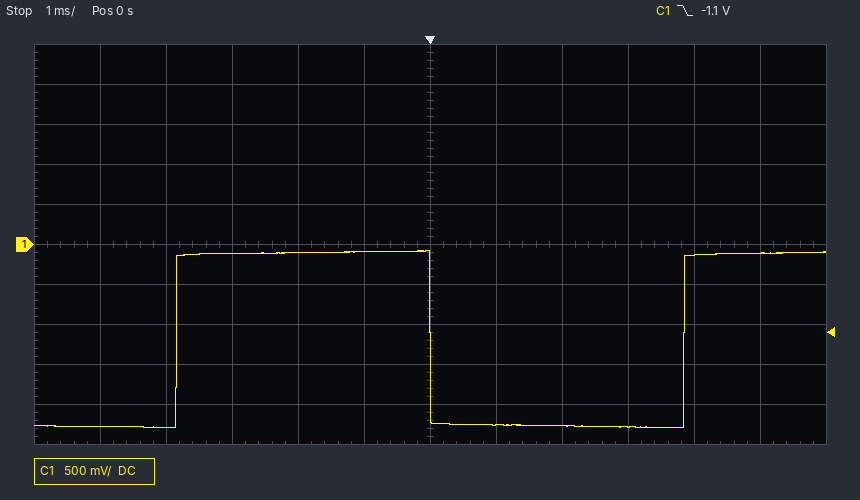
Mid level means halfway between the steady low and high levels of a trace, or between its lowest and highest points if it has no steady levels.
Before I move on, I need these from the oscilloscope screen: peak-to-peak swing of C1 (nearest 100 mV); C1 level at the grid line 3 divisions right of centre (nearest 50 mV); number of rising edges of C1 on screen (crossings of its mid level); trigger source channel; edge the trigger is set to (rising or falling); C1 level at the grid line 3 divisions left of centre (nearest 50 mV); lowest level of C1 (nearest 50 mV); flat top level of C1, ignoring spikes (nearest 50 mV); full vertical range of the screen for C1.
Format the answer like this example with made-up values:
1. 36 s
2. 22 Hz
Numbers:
1. 2.20 V
2. -2.30 V
3. 2
4. C1
5. falling
6. -100 mV
7. -2.30 V
8. -100 mV
9. 5 V
